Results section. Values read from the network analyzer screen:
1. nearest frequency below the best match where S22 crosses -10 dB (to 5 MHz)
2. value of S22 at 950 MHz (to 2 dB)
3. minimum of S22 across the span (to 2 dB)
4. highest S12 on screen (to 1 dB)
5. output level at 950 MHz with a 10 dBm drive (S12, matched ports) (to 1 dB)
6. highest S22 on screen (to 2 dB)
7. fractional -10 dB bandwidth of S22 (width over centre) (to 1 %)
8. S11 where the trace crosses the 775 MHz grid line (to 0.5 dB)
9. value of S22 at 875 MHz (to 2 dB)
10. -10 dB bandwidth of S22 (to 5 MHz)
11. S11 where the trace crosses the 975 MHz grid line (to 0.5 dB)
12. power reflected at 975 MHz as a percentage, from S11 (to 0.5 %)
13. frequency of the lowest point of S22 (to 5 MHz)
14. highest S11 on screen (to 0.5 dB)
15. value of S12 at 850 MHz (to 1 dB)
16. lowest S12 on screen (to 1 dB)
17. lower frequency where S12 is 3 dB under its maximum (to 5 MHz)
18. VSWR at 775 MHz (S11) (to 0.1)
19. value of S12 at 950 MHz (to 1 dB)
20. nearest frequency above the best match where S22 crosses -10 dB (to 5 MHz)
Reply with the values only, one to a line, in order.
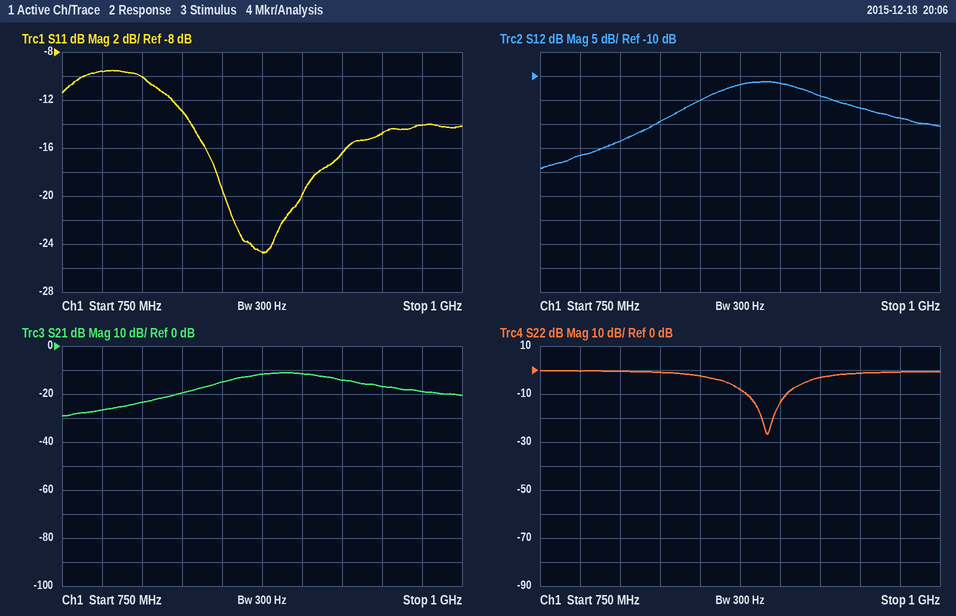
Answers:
880 MHz
-2 dB
-26 dB
-11 dB
-7 dBm
0 dB
3 %
-9.5 dB
-8 dB
25 MHz
-14.0 dB
4.0 %
890 MHz
-9.5 dB
-15 dB
-29 dB
855 MHz
2.0
-17 dB
905 MHz
